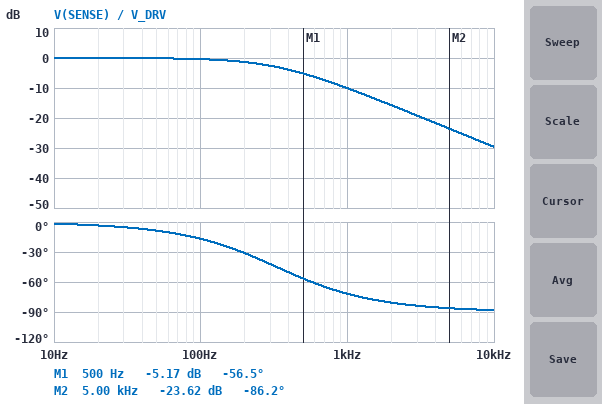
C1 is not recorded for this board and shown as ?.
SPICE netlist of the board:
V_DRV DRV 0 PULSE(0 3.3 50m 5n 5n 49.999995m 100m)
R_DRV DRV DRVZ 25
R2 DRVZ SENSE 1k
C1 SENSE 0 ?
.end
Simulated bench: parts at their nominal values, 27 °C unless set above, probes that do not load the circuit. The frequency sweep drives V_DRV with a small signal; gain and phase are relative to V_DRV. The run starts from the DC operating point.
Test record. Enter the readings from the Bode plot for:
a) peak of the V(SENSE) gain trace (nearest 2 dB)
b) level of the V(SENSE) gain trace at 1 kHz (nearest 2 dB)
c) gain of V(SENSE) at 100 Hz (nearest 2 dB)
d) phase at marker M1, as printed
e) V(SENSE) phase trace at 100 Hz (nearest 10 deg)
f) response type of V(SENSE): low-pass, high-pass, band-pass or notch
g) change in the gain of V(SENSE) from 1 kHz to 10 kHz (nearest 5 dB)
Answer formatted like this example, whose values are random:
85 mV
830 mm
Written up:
0 dB
-10 dB
0 dB
-56.5 deg
-20 deg
low-pass
-20 dB
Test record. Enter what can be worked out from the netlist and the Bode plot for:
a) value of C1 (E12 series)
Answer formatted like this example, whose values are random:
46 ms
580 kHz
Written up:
470 nF
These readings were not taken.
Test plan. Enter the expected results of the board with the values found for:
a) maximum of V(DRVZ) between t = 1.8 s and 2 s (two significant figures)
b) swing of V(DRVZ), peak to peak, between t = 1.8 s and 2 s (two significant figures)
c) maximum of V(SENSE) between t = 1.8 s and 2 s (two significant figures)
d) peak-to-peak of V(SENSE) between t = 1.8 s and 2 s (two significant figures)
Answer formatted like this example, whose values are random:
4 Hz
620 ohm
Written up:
3.3 V
3.3 V
3.3 V
3.3 V
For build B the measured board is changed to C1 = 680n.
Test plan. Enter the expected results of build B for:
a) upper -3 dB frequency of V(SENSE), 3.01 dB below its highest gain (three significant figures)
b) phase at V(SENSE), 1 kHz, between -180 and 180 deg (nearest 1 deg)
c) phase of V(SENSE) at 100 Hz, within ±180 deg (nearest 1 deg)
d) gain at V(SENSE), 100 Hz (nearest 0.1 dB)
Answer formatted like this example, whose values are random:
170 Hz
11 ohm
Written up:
228 Hz
-77 deg
-24 deg
-0.8 dB
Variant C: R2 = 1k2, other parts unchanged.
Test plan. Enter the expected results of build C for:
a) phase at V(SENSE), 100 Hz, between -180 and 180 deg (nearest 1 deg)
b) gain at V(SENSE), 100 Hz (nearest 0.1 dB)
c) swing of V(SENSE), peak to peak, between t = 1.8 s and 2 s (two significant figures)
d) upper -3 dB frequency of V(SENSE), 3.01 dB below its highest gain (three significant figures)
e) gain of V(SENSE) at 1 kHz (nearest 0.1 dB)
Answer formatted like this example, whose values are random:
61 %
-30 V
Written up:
-20 deg
-0.5 dB
3.3 V
276 Hz
-11.5 dB
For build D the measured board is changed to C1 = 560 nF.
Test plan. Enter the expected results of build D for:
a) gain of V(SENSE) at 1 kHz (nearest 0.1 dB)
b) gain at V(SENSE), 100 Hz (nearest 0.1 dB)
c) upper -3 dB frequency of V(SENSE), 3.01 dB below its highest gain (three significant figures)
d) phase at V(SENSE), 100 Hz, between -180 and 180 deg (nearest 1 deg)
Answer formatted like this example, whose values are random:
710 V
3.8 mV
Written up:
-11.5 dB
-0.5 dB
277 Hz
-20 deg
